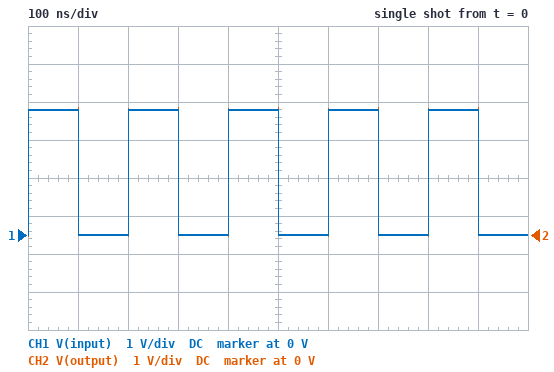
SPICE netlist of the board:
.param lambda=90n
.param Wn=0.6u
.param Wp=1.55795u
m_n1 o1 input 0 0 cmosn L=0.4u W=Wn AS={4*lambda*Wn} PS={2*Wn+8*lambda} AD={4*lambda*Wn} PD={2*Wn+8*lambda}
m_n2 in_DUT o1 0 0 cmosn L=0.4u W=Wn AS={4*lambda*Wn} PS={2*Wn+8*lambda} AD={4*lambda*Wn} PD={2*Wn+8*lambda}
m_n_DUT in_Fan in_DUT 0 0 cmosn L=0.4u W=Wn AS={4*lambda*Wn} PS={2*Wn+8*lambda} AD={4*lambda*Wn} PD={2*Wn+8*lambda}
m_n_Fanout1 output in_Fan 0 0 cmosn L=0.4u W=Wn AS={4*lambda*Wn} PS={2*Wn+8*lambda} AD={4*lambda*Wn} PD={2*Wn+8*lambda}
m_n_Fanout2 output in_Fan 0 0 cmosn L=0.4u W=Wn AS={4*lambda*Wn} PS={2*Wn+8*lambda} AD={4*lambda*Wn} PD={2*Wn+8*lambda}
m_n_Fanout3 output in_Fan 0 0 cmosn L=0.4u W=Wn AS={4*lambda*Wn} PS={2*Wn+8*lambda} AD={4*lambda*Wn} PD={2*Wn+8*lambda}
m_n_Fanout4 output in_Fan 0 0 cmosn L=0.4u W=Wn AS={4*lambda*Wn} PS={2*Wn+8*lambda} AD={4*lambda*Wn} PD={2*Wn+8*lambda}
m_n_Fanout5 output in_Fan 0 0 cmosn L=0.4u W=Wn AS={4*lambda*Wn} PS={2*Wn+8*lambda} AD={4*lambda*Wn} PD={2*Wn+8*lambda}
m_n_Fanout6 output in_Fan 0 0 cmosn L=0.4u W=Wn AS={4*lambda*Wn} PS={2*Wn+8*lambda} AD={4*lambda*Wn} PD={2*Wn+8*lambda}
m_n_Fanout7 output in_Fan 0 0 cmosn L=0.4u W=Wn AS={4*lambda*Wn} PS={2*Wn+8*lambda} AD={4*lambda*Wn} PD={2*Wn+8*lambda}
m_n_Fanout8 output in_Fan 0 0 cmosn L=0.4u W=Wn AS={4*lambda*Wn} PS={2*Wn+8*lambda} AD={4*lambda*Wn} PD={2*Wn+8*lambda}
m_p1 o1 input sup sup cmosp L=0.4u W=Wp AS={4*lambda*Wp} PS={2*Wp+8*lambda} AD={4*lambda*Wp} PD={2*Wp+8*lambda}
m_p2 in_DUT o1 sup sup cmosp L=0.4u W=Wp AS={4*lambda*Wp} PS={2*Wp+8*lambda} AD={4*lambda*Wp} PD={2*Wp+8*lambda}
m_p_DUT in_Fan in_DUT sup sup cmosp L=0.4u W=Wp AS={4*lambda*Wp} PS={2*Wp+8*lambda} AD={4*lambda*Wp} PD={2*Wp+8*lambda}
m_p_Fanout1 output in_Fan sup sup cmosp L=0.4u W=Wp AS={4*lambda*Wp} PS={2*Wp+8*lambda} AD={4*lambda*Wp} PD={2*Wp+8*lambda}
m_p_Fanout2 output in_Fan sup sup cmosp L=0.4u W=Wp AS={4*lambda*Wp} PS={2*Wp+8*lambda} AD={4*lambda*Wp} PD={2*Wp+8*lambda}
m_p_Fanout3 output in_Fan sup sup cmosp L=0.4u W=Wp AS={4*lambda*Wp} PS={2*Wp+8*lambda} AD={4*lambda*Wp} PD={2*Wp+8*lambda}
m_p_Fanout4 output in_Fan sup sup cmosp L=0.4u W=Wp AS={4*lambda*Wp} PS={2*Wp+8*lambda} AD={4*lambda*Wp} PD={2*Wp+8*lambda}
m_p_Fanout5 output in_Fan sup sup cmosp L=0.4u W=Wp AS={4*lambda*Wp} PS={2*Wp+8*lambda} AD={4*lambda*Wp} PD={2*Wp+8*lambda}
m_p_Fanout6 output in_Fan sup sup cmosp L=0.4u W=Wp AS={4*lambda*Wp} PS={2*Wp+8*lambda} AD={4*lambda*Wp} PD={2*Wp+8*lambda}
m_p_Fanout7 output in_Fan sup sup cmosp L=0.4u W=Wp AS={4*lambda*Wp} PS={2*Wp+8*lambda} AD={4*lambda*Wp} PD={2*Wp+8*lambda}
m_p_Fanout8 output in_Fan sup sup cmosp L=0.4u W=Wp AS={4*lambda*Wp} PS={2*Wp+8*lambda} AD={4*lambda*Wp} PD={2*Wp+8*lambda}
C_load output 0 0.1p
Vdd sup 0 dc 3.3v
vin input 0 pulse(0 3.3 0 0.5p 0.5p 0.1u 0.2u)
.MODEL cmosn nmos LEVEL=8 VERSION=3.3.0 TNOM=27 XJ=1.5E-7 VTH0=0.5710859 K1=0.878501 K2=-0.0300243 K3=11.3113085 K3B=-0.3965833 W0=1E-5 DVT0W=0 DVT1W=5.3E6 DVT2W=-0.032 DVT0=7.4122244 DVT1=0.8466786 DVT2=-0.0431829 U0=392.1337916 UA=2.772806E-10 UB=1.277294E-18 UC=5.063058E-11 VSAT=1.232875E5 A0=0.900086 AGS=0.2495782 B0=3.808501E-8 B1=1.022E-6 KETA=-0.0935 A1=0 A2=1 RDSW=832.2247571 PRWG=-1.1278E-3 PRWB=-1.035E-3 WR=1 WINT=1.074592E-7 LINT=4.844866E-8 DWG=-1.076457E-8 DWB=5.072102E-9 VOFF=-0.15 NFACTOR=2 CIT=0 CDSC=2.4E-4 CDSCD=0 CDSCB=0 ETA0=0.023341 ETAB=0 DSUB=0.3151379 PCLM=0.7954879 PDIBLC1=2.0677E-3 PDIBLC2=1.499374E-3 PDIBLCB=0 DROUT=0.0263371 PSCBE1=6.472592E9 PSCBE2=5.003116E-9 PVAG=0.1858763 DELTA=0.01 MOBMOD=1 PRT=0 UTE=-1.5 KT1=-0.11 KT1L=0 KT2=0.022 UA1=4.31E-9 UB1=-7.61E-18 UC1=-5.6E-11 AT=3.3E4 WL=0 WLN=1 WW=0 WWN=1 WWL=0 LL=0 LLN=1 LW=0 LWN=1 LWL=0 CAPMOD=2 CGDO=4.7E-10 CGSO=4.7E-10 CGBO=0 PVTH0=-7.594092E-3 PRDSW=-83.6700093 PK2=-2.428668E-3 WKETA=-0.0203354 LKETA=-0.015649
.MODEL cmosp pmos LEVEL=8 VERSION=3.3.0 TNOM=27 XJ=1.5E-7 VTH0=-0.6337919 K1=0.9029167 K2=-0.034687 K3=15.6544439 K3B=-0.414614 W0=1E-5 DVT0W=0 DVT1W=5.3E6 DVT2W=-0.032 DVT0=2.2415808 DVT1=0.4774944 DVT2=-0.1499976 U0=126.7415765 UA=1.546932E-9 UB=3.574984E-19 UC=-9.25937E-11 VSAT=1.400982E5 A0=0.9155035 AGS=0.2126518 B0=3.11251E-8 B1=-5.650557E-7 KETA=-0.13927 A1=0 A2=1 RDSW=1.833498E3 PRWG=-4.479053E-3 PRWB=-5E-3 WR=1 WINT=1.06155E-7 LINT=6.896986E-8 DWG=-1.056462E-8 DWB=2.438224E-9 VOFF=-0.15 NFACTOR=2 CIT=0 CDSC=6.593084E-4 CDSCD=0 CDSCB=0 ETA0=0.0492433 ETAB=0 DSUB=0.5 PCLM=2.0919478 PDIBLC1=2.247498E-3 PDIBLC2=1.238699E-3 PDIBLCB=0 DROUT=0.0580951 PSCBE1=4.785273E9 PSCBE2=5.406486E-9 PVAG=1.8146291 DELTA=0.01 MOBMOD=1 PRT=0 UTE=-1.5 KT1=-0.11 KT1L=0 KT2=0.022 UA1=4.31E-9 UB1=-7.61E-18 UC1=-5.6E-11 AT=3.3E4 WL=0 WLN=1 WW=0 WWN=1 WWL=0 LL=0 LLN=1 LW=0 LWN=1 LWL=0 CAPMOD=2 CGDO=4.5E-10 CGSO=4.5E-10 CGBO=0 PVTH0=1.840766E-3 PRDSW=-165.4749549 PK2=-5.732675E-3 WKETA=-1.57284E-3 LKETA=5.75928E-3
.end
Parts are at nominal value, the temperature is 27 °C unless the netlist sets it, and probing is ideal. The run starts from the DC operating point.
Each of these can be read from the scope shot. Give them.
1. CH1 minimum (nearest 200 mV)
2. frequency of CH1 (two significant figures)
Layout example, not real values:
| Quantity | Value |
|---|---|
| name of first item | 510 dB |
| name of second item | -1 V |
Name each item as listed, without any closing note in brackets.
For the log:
| Quantity | Value |
|---|---|
| CH1 minimum | 0 V |
| frequency of CH1 | 5.0 MHz |
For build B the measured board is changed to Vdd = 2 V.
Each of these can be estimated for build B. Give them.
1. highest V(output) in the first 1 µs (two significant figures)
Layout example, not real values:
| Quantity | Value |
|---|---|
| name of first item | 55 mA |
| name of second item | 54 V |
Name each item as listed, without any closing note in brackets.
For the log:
| Quantity | Value |
|---|---|
| highest V(output) in the first 1 µs | 2.0 V |
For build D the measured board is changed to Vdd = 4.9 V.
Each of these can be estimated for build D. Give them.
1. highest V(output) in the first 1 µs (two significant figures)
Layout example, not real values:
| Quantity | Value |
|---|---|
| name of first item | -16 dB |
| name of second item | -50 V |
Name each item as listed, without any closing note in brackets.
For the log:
| Quantity | Value |
|---|---|
| highest V(output) in the first 1 µs | 5.0 V |
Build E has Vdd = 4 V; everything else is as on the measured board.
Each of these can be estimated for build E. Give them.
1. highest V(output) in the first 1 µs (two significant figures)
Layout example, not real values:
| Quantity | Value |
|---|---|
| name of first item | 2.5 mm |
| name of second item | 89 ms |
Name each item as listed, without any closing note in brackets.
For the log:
| Quantity | Value |
|---|---|
| highest V(output) in the first 1 µs | 4.1 V |
